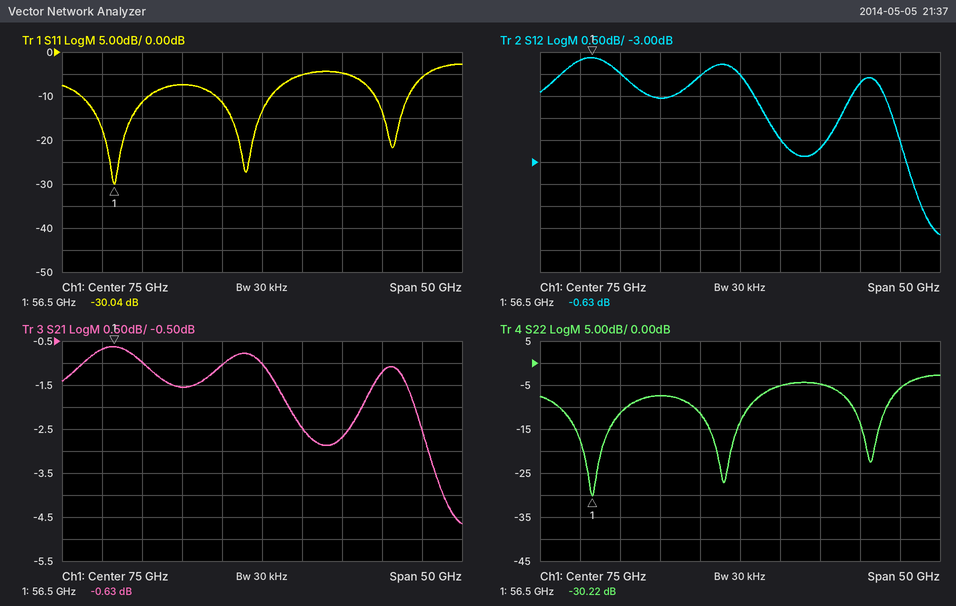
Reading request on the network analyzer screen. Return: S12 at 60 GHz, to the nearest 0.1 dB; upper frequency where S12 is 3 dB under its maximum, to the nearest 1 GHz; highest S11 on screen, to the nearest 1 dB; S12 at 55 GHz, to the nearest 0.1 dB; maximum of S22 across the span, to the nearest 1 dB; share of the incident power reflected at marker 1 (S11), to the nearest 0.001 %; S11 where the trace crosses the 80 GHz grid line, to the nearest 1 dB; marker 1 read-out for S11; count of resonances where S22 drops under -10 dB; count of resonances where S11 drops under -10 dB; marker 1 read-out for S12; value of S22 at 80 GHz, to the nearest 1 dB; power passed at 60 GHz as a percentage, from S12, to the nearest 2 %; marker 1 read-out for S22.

-1.0 dB
97 GHz
-3 dB
-0.7 dB
-3 dB
0.099 %
-5 dB
-30.04 dB
3
3
-0.63 dB
-5 dB
80 %
-30.22 dB
